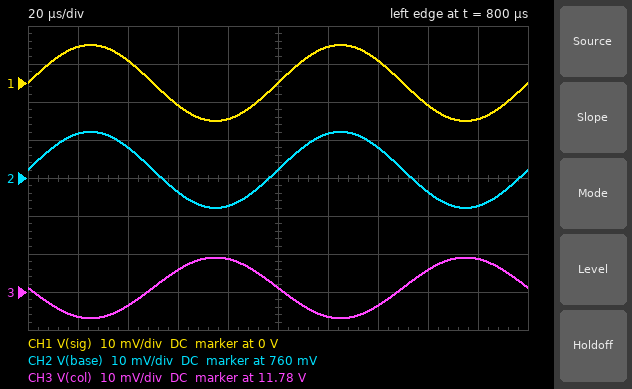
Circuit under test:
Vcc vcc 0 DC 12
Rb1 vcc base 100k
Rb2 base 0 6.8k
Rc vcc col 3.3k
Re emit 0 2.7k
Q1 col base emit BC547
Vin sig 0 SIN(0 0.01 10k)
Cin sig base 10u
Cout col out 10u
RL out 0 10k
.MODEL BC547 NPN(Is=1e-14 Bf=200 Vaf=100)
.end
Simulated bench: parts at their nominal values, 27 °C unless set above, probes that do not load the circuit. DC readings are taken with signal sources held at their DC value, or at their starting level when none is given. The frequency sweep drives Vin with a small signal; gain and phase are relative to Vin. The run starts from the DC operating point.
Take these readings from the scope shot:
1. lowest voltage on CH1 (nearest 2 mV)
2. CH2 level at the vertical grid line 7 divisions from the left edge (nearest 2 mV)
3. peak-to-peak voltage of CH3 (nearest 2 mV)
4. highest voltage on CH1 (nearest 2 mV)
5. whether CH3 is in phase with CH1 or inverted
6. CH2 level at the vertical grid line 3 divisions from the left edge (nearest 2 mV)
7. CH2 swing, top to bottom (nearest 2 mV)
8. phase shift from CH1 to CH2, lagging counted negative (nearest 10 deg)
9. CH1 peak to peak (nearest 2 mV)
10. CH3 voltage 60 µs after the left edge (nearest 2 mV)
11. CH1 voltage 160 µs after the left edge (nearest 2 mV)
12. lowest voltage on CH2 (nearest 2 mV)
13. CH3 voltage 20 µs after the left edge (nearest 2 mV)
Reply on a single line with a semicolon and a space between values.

-10 mV; 768 mV; 16 mV; 10 mV; inverted; 756 mV; 20 mV; 0 deg; 20 mV; 11.786 V; -6 mV; 752 mV; 11.774 V
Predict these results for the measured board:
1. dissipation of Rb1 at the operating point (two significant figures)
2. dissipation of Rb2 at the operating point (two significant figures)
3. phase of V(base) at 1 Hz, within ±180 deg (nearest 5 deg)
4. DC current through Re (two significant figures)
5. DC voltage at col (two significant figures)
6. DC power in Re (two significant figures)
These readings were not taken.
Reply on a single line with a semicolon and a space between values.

1.3 mW; 85 µW; 70 deg; 67 µA; 12 V; 12 µW
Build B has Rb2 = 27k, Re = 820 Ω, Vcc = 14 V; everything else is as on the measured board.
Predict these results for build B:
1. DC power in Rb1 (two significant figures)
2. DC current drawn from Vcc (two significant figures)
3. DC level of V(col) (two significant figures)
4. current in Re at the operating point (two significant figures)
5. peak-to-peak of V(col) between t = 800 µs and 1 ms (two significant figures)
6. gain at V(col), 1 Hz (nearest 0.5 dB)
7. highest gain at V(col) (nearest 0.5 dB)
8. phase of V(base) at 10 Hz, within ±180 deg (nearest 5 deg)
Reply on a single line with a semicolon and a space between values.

1.3 mW; 2.6 mA; 5.8 V; 2.5 mA; 59 mV; 8.5 dB; 9.5 dB; 5 deg
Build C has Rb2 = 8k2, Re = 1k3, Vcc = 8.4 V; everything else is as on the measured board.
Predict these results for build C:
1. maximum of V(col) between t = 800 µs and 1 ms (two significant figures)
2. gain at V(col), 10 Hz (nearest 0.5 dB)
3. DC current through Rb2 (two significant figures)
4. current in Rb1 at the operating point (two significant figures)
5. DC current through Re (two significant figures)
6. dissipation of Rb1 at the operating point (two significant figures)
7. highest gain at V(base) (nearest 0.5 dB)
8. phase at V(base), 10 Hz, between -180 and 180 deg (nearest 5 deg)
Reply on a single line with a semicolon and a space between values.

8.3 V; 2.5 dB; 77 µA; 78 µA; 47 µA; 600 µW; 0 dB; 10 deg
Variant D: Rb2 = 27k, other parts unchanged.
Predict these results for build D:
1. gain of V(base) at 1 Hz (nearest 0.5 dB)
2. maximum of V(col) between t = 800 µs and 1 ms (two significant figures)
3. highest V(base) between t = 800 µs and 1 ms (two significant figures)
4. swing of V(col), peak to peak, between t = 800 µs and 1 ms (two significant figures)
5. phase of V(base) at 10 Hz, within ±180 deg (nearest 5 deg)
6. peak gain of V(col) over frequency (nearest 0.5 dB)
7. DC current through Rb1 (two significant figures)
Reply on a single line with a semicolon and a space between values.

-2.0 dB; 9.8 V; 2.5 V; 18 mV; 5 deg; -0.5 dB; 95 µA
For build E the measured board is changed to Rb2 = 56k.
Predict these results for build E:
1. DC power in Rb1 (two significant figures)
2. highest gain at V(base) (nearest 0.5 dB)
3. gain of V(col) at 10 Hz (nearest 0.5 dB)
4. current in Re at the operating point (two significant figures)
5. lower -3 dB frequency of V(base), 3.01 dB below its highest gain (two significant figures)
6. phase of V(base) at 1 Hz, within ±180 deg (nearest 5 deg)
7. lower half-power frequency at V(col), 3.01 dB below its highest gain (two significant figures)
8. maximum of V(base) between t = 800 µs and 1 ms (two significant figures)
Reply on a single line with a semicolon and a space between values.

630 µW; 0 dB; -1.0 dB; 1.3 mA; 470 mHz; 25 deg; 350 mHz; 4.1 V
